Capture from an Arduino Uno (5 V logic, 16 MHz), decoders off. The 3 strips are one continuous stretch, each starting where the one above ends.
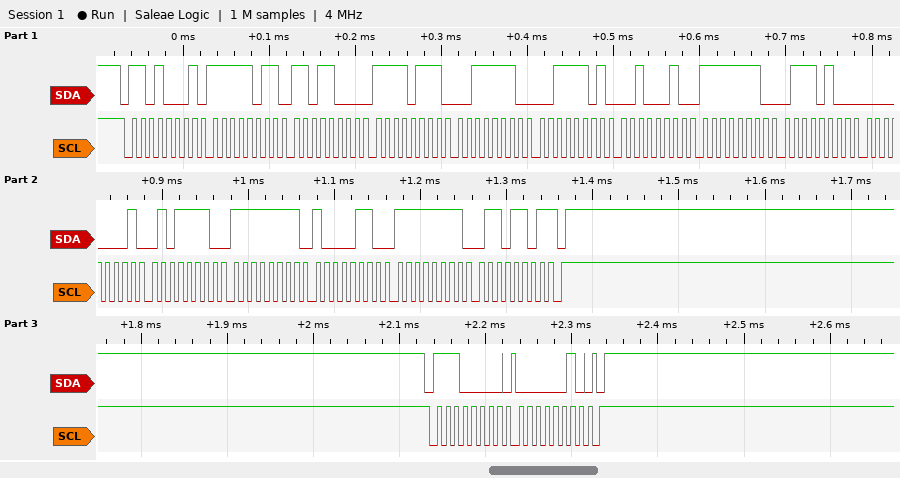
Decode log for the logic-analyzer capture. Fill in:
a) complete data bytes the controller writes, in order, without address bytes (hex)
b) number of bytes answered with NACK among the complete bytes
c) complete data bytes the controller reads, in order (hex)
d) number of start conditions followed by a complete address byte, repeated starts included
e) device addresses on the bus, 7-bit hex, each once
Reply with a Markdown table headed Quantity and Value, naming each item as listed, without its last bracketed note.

| Quantity | Value |
|---|---|
| complete data bytes the controller writes, in order, without address bytes | 02 |
| number of bytes answered with NACK among the complete bytes | 1 |
| complete data bytes the controller reads, in order | FB D8 F7 3E 3D 22 FE 74 01 5E FF 86 FF 6D |
| number of start conditions followed by a complete address byte, repeated starts included | 2 |
| device addresses on the bus, 7-bit hex, each once | 0x68 0x70 |
